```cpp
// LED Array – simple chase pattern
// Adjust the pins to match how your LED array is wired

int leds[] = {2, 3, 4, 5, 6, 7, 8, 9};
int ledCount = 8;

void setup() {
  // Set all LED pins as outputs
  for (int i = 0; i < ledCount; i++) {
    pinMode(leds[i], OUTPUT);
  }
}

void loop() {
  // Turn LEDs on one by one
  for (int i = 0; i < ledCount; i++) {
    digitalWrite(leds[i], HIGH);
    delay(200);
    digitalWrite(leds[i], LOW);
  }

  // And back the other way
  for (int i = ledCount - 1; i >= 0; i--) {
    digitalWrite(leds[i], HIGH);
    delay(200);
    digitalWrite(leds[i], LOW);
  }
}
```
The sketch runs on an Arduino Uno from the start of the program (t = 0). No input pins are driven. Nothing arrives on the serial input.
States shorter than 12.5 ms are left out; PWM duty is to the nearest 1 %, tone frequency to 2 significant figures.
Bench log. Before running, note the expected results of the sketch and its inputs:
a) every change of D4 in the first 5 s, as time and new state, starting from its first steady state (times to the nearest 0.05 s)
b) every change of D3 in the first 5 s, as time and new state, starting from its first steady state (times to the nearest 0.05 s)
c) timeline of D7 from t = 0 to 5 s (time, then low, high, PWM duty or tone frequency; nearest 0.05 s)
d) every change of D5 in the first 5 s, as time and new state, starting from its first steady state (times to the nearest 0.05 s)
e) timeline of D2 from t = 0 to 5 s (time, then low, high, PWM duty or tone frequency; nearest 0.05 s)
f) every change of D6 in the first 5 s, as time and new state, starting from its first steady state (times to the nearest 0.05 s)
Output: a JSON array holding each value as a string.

["0 s low; 0.4 s high; 0.6 s low; 2.6 s high; 2.8 s low; 3.6 s high; 3.8 s low", "0 s low; 0.2 s high; 0.4 s low; 2.8 s high; 3 s low; 3.4 s high; 3.6 s low", "0 s low; 1 s high; 1.2 s low; 2 s high; 2.2 s low; 4.2 s high; 4.4 s low", "0 s low; 0.6 s high; 0.8 s low; 2.4 s high; 2.6 s low; 3.8 s high; 4 s low", "0 s high; 0.2 s low; 3 s high; 3.4 s low", "0 s low; 0.8 s high; 1 s low; 2.2 s high; 2.4 s low; 4 s high; 4.2 s low"]
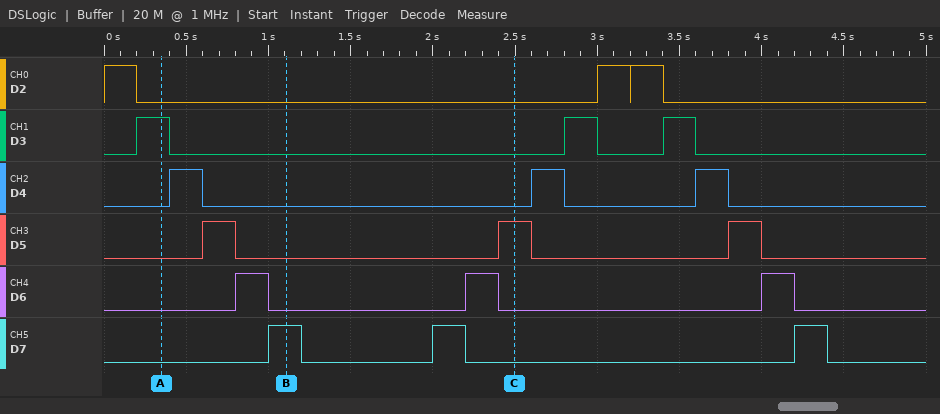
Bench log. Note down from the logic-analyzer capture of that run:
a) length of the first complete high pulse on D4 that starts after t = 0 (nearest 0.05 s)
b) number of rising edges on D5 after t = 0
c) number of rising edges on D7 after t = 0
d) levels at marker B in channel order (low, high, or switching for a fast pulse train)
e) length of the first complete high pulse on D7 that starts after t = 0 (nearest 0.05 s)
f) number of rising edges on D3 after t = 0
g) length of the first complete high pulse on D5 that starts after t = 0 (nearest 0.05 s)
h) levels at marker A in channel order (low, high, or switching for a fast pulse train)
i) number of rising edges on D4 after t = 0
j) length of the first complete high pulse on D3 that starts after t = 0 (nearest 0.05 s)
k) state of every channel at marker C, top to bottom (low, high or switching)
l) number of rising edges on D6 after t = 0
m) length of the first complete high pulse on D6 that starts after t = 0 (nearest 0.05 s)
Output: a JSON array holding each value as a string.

["0.20 s", "3", "3", "D2 low, D3 low, D4 low, D5 low, D6 low, D7 high", "0.20 s", "3", "0.20 s", "D2 low, D3 high, D4 low, D5 low, D6 low, D7 low", "3", "0.20 s", "D2 low, D3 low, D4 low, D5 high, D6 low, D7 low", "3", "0.20 s"]
